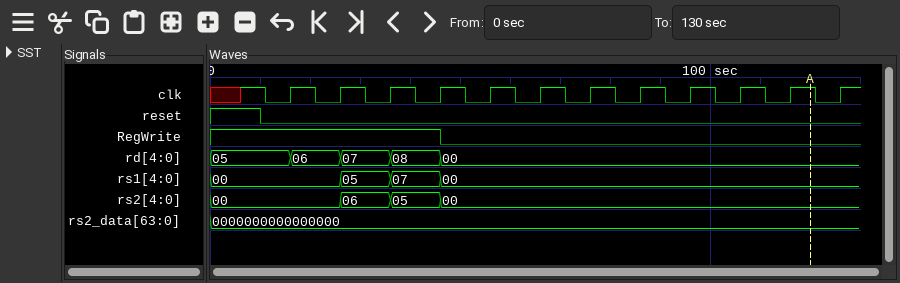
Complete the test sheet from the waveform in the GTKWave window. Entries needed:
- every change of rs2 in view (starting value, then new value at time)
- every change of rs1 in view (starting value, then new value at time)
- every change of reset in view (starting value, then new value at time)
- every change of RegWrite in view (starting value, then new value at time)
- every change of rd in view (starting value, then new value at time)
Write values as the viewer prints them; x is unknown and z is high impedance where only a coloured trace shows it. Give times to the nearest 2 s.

00, 06 at 26 s, 05 at 36 s, 00 at 46 s
00, 05 at 26 s, 07 at 36 s, 00 at 46 s
1, 0 at 10 s
1, 0 at 46 s
05, 06 at 16 s, 07 at 26 s, 08 at 36 s, 00 at 46 s
